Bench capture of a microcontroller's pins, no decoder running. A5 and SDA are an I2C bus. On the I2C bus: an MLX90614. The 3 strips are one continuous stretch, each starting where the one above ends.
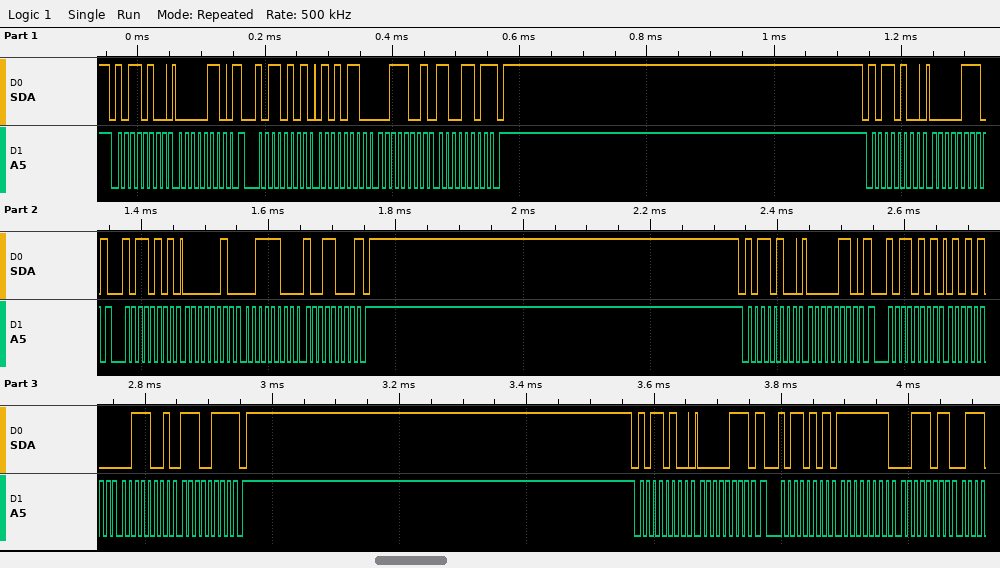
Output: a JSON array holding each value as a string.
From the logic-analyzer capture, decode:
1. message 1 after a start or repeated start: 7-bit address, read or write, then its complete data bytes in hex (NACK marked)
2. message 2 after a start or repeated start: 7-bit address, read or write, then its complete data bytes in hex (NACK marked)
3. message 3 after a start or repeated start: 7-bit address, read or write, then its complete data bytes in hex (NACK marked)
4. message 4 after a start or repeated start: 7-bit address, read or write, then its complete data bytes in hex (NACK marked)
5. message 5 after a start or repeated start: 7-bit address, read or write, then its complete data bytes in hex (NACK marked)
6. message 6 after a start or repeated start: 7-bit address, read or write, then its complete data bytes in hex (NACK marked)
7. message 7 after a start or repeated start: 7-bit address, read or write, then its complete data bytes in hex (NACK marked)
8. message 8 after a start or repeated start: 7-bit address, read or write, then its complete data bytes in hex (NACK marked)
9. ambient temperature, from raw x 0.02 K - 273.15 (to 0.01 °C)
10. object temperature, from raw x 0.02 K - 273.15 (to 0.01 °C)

["0x5A write: 06", "0x5A read: 56 39 CD NACK", "0x5A write: 07", "0x5A read: 02 3C 98 NACK", "0x5A write: 06", "0x5A read: 54 39 E7 NACK", "0x5A write: 07", "0x5A read: FF 3B", "20.41 °C", "34.09 °C"]
